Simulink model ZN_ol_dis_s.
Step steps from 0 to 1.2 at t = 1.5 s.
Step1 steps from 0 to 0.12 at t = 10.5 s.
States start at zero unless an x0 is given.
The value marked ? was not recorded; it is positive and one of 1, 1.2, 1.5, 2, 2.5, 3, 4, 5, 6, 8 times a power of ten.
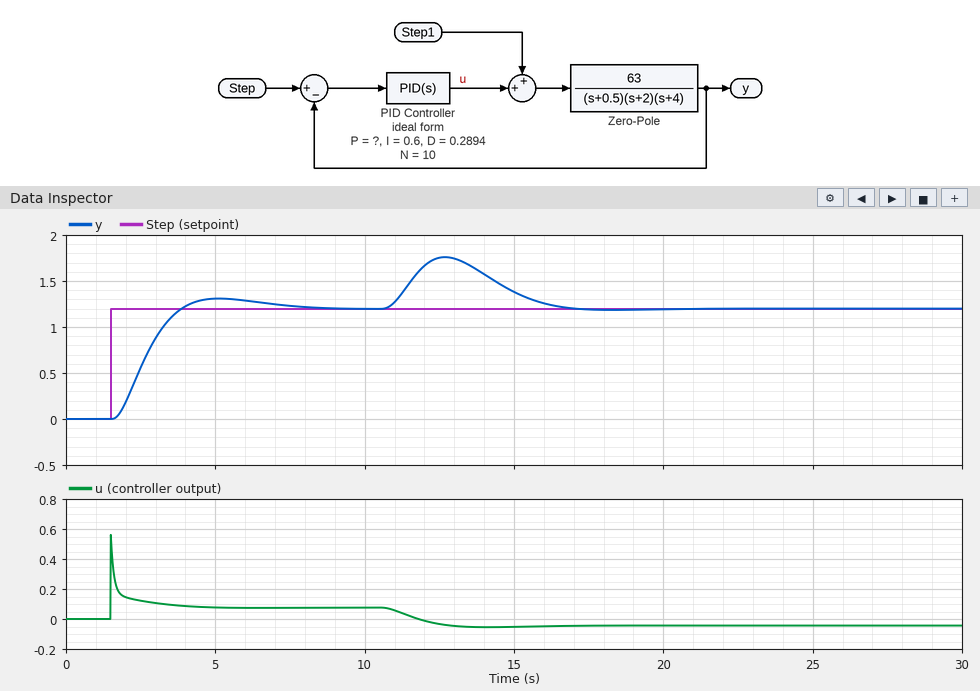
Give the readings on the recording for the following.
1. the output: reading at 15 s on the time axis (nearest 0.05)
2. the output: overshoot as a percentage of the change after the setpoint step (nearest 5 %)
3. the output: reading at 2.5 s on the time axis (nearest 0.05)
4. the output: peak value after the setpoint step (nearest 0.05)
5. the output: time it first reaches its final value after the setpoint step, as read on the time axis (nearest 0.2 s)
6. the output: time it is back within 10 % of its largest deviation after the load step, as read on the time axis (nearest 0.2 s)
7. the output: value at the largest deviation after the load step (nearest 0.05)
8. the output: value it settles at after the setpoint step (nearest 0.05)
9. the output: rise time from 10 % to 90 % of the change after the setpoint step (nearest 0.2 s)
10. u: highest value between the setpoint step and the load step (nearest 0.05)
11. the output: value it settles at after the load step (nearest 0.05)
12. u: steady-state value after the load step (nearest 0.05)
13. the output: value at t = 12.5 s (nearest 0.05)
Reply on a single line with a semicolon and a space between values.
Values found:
1.40; 10 %; 0.55; 1.30; 3.8 s; 16.0 s; 1.75; 1.20; 1.6 s; 0.55; 1.20; -0.05; 1.75
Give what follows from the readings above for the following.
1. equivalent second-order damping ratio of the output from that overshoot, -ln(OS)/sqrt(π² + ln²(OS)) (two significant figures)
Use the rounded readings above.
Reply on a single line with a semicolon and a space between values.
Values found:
0.59
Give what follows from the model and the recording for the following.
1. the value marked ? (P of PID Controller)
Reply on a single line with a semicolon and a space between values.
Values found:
0.12
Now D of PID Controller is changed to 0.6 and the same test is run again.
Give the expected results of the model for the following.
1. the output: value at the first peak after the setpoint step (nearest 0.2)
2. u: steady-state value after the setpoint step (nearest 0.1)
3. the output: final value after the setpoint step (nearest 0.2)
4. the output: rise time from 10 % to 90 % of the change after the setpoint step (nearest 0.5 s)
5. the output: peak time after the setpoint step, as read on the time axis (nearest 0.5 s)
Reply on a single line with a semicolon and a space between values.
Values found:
1.2; 0.1; 1.2; 2.0 s; 6.5 s
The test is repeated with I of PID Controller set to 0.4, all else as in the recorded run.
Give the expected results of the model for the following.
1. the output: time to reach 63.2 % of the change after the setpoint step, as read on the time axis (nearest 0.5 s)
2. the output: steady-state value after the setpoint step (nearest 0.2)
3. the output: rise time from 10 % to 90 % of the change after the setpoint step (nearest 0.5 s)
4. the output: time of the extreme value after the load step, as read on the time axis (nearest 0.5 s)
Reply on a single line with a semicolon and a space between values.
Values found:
3.0 s; 1.2; 2.0 s; 13.0 s
